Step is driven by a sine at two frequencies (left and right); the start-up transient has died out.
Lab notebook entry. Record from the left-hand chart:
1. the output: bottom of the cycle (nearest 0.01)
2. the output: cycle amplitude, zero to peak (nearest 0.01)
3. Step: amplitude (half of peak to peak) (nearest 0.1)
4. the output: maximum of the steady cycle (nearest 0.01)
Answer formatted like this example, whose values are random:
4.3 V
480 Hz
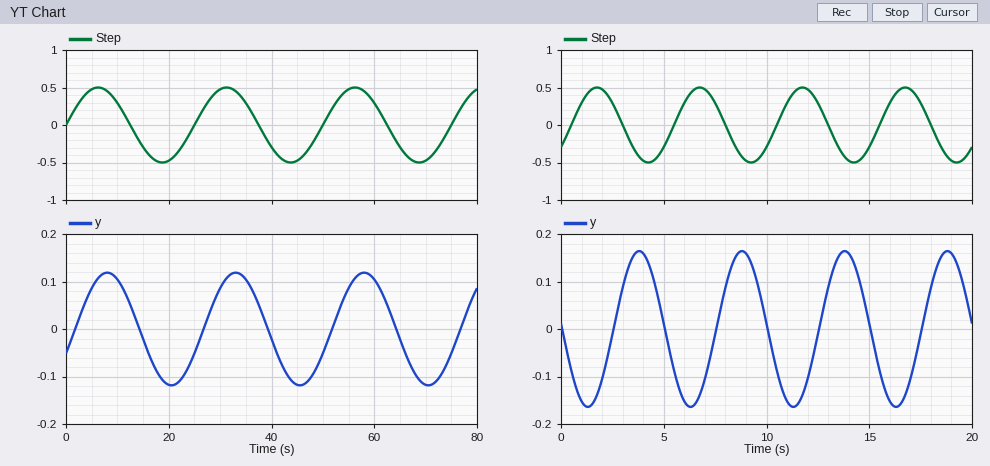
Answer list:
-0.12
0.12
0.5
0.12
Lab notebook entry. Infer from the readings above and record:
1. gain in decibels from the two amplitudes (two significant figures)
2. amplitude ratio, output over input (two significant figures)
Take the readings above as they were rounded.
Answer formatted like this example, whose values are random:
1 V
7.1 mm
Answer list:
-12 dB
0.24
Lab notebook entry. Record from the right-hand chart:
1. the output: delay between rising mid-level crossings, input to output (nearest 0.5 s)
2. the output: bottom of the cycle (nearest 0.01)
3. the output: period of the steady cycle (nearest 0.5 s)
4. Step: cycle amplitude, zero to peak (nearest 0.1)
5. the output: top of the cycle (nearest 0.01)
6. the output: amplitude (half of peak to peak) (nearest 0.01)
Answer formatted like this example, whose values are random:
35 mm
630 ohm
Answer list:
2.0 s
-0.16
5.0 s
0.5
0.16
0.16
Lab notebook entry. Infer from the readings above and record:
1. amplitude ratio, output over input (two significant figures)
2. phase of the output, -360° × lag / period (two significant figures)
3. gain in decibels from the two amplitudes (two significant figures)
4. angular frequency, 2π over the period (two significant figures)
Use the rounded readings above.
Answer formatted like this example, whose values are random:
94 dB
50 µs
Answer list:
0.32
-140°
-9.9 dB
1.3 rad/s
